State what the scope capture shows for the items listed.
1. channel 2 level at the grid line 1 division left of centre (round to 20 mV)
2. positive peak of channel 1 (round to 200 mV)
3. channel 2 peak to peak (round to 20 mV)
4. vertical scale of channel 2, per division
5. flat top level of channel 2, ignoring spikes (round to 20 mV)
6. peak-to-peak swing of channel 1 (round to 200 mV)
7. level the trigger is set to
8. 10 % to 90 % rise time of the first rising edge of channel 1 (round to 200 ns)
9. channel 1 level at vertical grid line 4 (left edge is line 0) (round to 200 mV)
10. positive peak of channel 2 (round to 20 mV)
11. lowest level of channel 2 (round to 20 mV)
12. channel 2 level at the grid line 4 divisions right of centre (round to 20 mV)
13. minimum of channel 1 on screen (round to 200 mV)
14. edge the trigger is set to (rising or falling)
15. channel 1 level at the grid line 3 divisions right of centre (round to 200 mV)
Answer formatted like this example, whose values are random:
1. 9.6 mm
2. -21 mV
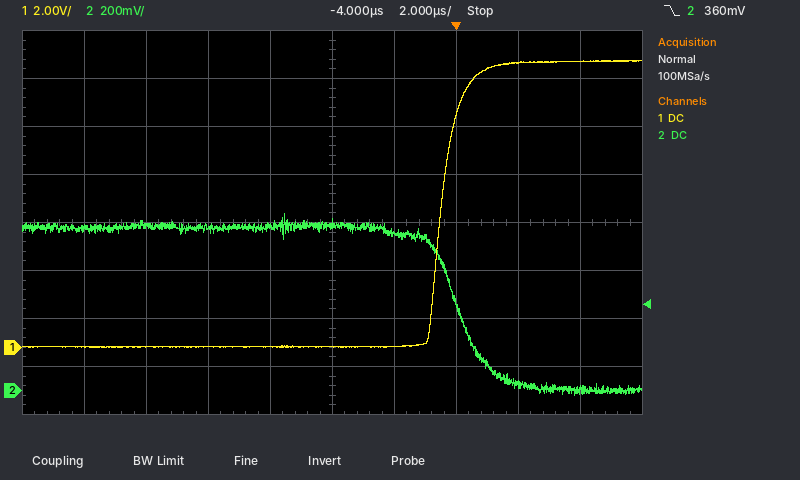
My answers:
1. 680 mV
2. 12.0 V
3. 760 mV
4. 200 mV
5. 680 mV
6. 12.0 V
7. 360 mV
8. 1.2 µs
9. 0.0 V
10. 740 mV
11. -20 mV
12. 0 mV
13. 0.0 V
14. falling
15. 11.8 V
